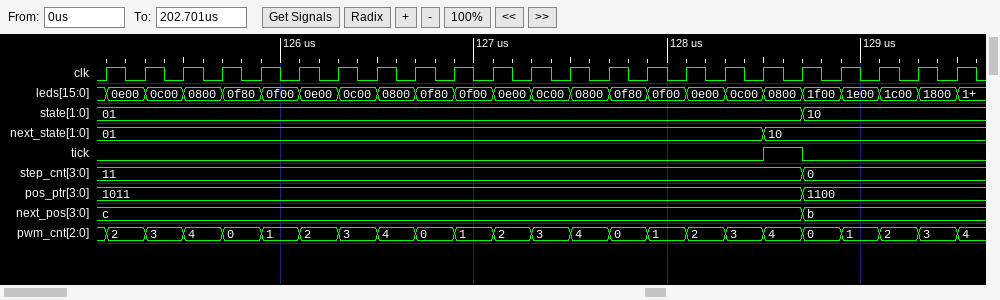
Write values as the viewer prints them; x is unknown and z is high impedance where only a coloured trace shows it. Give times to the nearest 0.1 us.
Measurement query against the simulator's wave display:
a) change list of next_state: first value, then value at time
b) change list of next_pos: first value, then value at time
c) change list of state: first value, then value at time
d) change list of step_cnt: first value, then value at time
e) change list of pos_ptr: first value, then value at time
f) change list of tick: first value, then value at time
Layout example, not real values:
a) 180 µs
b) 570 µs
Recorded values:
a) 01, 10 at 128.5 us
b) c, b at 128.7 us
c) 01, 10 at 128.7 us
d) 11, 0 at 128.7 us
e) 1011, 1100 at 128.7 us
f) 0, 1 at 128.5 us, 0 at 128.7 us
